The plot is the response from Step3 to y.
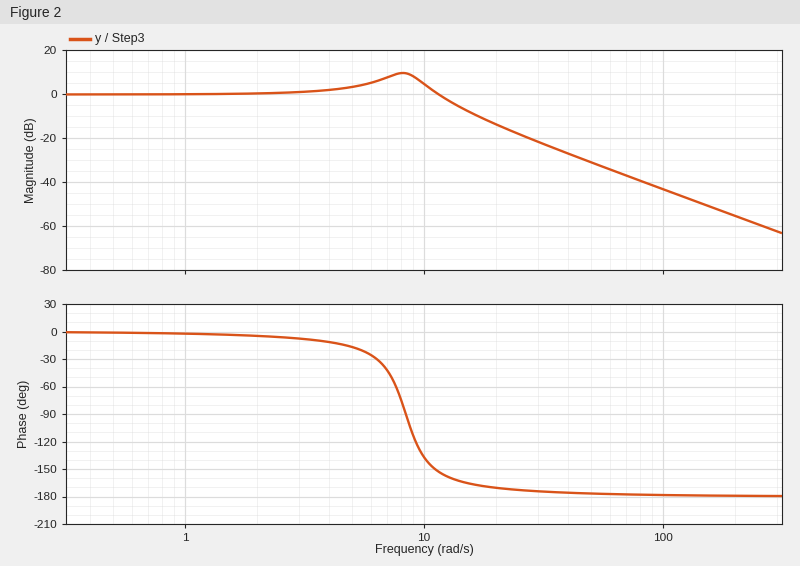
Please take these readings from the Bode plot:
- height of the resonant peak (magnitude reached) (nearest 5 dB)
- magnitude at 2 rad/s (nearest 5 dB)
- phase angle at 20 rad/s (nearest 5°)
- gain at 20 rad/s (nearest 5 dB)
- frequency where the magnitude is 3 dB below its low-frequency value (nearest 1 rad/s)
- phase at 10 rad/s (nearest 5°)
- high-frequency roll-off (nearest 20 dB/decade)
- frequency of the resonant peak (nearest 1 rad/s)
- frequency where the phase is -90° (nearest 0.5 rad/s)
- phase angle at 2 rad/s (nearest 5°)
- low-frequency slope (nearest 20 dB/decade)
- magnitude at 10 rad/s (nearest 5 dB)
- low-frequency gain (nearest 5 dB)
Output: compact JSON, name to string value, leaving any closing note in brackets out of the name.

{"height of the resonant peak (magnitude reached)": "10 dB", "magnitude at 2 rad/s": "0 dB", "phase angle at 20 rad/s": "-170°", "gain at 20 rad/s": "-15 dB", "frequency where the magnitude is 3 dB below its low-frequency value": "13 rad/s", "phase at 10 rad/s": "-135°", "high-frequency roll-off": "-40 dB/decade", "frequency of the resonant peak": "8 rad/s", "frequency where the phase is -90°": "8.5 rad/s", "phase angle at 2 rad/s": "-5°", "low-frequency slope": "0 dB/decade", "magnitude at 10 rad/s": "5 dB", "low-frequency gain": "0 dB"}
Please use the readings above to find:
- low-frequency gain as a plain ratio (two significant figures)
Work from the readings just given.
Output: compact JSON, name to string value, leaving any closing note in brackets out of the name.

{"low-frequency gain as a plain ratio": "1.0"}
